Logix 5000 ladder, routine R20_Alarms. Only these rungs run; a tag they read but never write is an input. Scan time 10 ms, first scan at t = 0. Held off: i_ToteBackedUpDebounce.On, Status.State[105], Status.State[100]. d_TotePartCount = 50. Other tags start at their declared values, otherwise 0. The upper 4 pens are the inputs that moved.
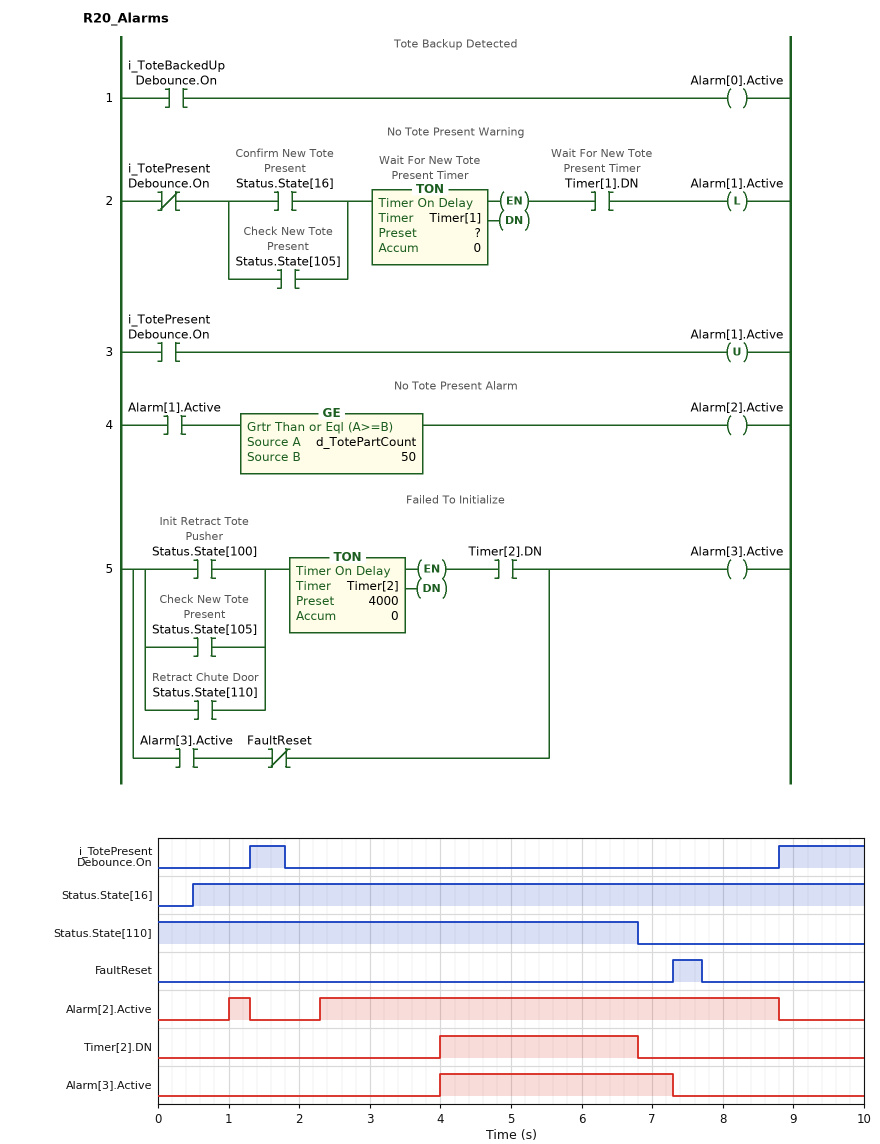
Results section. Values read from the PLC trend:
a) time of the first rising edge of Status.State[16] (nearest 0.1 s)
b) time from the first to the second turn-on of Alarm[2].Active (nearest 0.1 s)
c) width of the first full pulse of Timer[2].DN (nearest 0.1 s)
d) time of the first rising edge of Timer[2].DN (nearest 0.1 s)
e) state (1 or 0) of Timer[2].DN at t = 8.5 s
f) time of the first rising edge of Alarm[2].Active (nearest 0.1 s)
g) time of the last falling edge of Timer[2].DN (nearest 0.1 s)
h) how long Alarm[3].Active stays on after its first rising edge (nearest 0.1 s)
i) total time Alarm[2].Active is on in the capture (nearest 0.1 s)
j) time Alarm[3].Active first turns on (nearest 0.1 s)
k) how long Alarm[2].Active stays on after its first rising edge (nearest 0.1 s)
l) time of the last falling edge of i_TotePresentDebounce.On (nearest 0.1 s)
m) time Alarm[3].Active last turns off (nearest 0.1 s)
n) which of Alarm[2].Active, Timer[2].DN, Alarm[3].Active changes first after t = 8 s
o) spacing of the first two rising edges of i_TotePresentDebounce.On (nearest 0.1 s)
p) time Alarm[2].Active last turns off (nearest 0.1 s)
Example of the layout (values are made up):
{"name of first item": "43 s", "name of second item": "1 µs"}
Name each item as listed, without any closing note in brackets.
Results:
{"time of the first rising edge of Status.State[16]": "0.5 s", "time from the first to the second turn-on of Alarm[2].Active": "1.3 s", "width of the first full pulse of Timer[2].DN": "2.8 s", "time of the first rising edge of Timer[2].DN": "4.0 s", "state (1 or 0) of Timer[2].DN at t = 8.5 s": "0", "time of the first rising edge of Alarm[2].Active": "1.0 s", "time of the last falling edge of Timer[2].DN": "6.8 s", "how long Alarm[3].Active stays on after its first rising edge": "3.3 s", "total time Alarm[2].Active is on in the capture": "6.8 s", "time Alarm[3].Active first turns on": "4.0 s", "how long Alarm[2].Active stays on after its first rising edge": "0.3 s", "time of the last falling edge of i_TotePresentDebounce.On": "1.8 s", "time Alarm[3].Active last turns off": "7.3 s", "which of Alarm[2].Active, Timer[2].DN, Alarm[3].Active changes first after t = 8 s": "Alarm[2].Active", "spacing of the first two rising edges of i_TotePresentDebounce.On": "7.5 s", "time Alarm[2].Active last turns off": "8.8 s"}
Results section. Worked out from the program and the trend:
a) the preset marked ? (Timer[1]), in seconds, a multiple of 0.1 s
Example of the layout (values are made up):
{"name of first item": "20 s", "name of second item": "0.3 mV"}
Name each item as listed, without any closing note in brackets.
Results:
{"the preset marked ? (Timer[1]), in seconds, a multiple of 0.1 s": "0.5 s"}
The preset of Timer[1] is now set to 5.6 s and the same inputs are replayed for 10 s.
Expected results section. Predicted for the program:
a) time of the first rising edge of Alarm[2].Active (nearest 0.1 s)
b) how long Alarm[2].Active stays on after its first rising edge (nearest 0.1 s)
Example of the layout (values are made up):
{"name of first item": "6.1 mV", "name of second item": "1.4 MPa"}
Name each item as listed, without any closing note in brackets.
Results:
{"time of the first rising edge of Alarm[2].Active": "7.4 s", "how long Alarm[2].Active stays on after its first rising edge": "1.4 s"}
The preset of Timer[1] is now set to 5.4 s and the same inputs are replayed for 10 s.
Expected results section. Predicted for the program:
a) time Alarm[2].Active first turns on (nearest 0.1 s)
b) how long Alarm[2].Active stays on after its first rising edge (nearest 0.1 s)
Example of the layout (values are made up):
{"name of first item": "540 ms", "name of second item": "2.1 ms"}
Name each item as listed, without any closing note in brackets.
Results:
{"time Alarm[2].Active first turns on": "7.2 s", "how long Alarm[2].Active stays on after its first rising edge": "1.6 s"}
